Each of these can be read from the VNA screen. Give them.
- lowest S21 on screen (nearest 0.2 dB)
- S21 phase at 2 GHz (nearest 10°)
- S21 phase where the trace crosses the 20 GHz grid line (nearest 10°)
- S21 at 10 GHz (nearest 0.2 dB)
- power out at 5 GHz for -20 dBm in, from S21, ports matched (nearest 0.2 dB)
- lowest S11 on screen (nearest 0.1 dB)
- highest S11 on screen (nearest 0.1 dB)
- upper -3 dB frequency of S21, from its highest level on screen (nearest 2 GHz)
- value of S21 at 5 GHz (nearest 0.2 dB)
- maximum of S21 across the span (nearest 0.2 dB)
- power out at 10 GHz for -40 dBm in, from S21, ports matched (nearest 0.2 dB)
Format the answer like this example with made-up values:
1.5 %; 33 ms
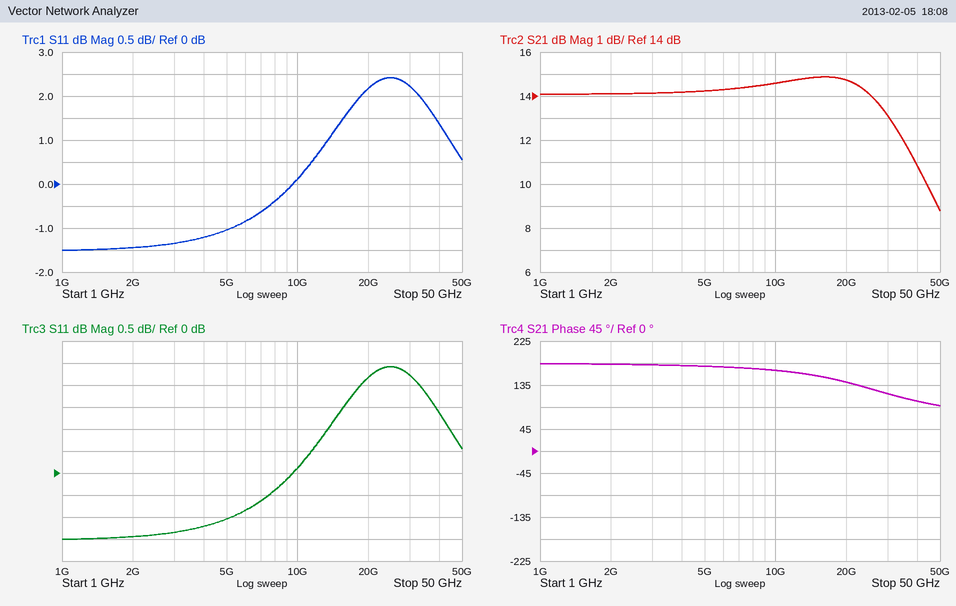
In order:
8.8 dB; 180°; 140°; 14.6 dB; -5.8 dBm; -1.5 dB; 2.4 dB; 36 GHz; 14.2 dB; 14.8 dB; -25.4 dBm
